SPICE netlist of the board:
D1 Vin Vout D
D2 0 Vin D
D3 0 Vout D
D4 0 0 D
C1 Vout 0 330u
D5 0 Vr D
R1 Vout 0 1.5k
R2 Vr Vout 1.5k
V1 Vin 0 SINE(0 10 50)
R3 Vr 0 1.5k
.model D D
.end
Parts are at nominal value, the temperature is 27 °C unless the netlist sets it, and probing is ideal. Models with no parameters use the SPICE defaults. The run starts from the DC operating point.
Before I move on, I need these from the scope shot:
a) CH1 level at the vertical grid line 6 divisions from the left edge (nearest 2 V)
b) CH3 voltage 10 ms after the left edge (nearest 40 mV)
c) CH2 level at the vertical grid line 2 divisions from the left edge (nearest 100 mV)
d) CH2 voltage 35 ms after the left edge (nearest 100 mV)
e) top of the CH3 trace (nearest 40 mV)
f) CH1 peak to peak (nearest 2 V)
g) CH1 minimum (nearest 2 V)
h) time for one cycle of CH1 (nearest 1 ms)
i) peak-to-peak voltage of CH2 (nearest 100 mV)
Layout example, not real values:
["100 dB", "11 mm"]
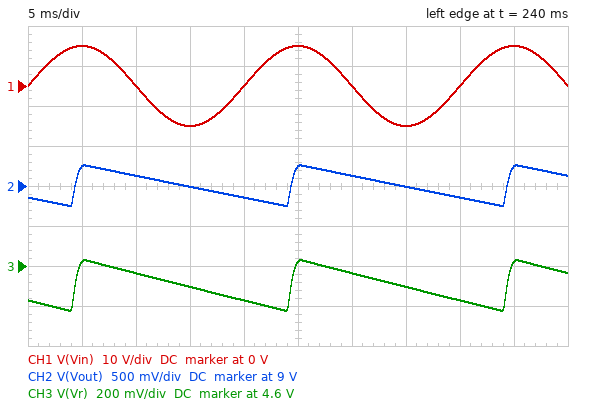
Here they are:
["0 V", "4.56 V", "9.1 V", "9.0 V", "4.64 V", "20 V", "-10 V", "20 ms", "500 mV"]
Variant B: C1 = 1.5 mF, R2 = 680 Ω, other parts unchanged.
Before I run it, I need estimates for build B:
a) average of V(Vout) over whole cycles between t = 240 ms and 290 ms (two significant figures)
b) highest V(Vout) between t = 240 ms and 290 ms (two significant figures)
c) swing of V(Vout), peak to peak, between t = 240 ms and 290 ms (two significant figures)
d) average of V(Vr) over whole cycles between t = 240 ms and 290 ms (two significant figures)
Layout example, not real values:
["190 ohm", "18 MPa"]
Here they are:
["9.2 V", "9.2 V", "130 mV", "6.3 V"]
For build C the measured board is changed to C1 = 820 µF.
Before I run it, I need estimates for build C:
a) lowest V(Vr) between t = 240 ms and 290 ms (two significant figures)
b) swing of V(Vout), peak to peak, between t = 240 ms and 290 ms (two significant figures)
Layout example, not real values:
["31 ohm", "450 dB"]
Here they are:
["4.5 V", "210 mV"]
